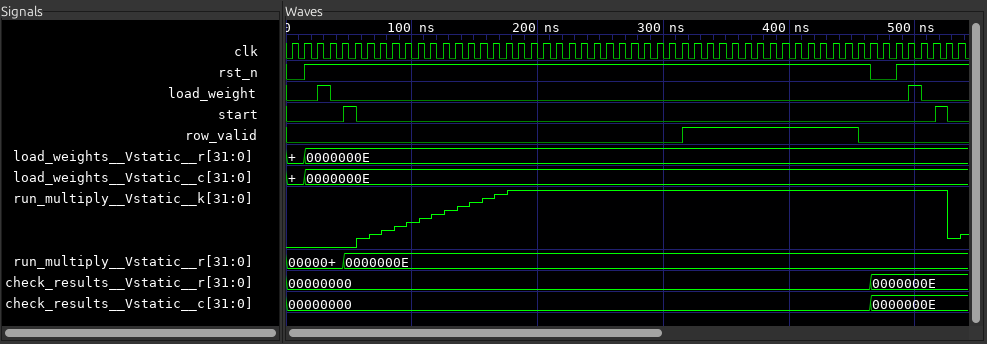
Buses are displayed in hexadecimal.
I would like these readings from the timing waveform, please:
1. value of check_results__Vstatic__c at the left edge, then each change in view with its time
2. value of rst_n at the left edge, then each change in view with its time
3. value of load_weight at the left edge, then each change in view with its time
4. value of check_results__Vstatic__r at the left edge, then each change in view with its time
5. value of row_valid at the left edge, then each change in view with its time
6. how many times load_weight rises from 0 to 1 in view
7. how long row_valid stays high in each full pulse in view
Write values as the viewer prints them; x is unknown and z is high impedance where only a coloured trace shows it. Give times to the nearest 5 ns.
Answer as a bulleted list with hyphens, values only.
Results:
- 00000000, 0000000E at 465 ns
- 0, 1 at 15 ns, 0 at 465 ns, 1 at 485 ns
- 0, 1 at 25 ns, 0 at 35 ns, 1 at 495 ns, 0 at 505 ns
- 00000000, 0000000E at 465 ns
- 0, 1 at 315 ns, 0 at 455 ns
- 2
- 140 ns
